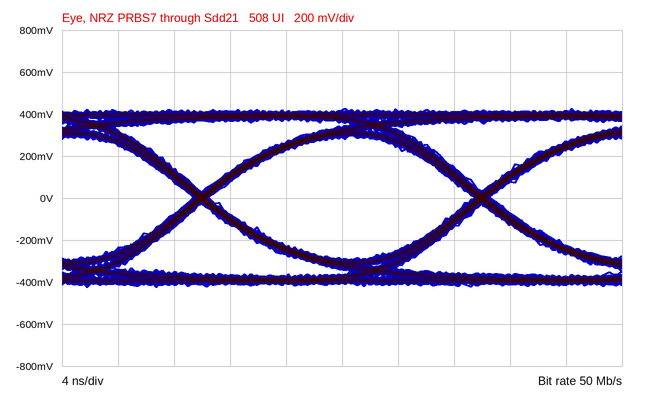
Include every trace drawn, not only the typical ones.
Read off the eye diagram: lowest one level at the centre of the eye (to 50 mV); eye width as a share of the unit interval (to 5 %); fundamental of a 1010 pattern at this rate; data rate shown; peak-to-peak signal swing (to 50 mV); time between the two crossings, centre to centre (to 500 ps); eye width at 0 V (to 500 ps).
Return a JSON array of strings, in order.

["300 mV", "95 %", "25 MHz", "50 Mb/s", "850 mV", "20.0 ns", "19.0 ns"]
